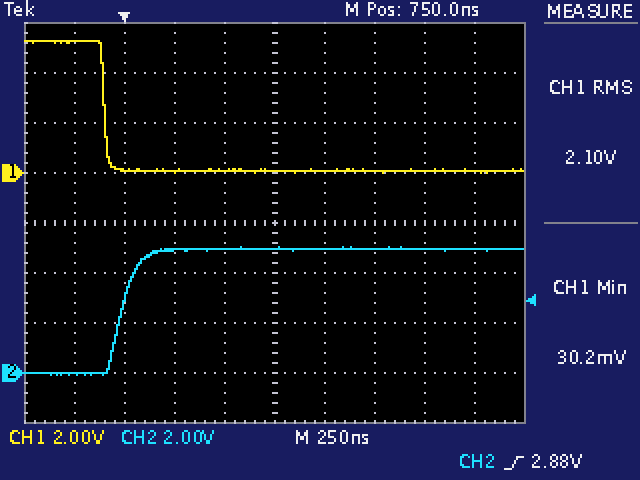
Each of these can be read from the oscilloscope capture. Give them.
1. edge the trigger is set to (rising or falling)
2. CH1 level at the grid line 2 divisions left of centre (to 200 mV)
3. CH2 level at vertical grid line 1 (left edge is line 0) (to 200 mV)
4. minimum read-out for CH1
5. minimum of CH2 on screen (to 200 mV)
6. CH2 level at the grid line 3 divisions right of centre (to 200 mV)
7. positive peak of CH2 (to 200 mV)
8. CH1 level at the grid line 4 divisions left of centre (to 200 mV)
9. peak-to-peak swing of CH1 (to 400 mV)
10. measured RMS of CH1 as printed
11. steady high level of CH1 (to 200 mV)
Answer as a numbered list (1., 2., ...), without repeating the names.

1. rising
2. 0.0 V
3. 0.0 V
4. 30.2 mV
5. 0.0 V
6. 5.0 V
7. 5.0 V
8. 5.2 V
9. 5.2 V
10. 2.10 V
11. 5.2 V
